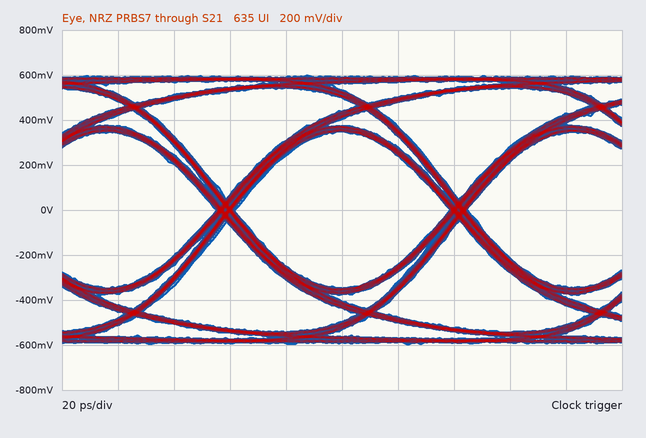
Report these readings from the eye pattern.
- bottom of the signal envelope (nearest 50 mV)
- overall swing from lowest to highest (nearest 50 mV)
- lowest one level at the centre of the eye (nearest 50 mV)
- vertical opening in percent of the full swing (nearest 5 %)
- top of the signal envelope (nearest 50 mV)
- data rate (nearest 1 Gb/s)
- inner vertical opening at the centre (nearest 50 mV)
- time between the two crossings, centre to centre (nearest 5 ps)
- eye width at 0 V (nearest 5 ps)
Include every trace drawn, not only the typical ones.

-600 mV
1.20 V
350 mV
60 %
600 mV
12 Gb/s
700 mV
85 ps
75 ps
